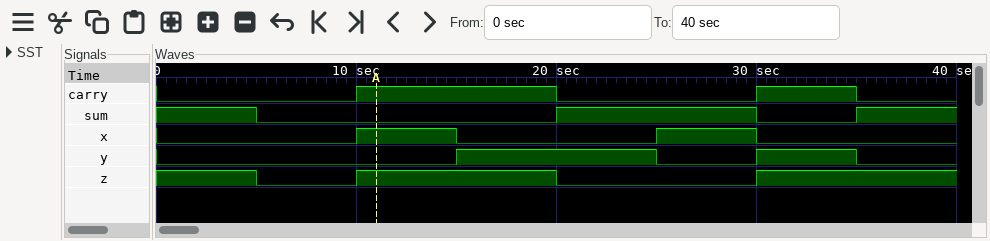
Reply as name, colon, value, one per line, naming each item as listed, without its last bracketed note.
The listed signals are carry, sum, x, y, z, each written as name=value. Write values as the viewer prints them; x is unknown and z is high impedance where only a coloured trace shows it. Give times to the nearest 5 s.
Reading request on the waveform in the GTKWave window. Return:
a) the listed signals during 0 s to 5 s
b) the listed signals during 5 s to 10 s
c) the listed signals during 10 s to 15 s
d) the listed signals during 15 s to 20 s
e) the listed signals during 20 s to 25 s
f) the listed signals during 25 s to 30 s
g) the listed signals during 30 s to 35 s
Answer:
the listed signals during 0 s to 5 s: carry=0, sum=1, x=0, y=0, z=1
the listed signals during 5 s to 10 s: carry=0, sum=0, x=0, y=0, z=0
the listed signals during 10 s to 15 s: carry=1, sum=0, x=1, y=0, z=1
the listed signals during 15 s to 20 s: carry=1, sum=0, x=0, y=1, z=1
the listed signals during 20 s to 25 s: carry=0, sum=1, x=0, y=1, z=0
the listed signals during 25 s to 30 s: carry=0, sum=1, x=1, y=0, z=0
the listed signals during 30 s to 35 s: carry=1, sum=0, x=0, y=1, z=1
